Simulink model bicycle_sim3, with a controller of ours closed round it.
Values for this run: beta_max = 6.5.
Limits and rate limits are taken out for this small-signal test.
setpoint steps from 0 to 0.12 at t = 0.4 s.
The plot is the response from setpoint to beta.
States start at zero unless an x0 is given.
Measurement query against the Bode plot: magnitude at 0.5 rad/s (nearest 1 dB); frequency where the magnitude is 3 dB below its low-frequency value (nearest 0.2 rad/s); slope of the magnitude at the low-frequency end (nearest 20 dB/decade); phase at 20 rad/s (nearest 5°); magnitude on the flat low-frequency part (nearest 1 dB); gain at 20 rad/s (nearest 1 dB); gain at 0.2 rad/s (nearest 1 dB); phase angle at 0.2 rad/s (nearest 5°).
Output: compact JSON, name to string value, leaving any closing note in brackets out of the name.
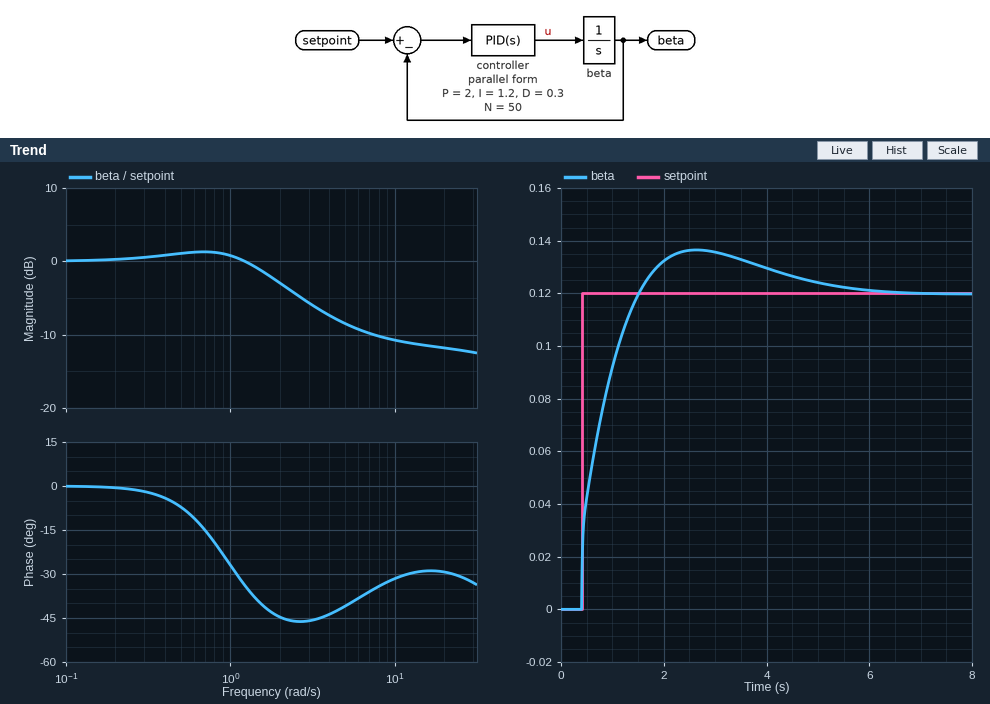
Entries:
{"magnitude at 0.5 rad/s": "1 dB", "frequency where the magnitude is 3 dB below its low-frequency value": "2.0 rad/s", "slope of the magnitude at the low-frequency end": "0 dB/decade", "phase at 20 rad/s": "-30°", "magnitude on the flat low-frequency part": "0 dB", "gain at 20 rad/s": "-12 dB", "gain at 0.2 rad/s": "0 dB", "phase angle at 0.2 rad/s": "0°"}
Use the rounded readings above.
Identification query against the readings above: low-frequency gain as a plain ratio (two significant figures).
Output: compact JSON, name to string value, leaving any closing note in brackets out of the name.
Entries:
{"low-frequency gain as a plain ratio": "1.0"}
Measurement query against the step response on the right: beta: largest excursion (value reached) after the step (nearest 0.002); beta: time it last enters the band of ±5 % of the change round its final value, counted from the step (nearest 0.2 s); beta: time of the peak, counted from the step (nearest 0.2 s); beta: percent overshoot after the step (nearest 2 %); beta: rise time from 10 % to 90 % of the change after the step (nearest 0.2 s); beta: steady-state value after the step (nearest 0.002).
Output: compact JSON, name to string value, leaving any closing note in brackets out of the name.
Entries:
{"beta: largest excursion (value reached) after the step": "0.136", "beta: time it last enters the band of ±5 % of the change round its final value, counted from the step": "4.2 s", "beta: time of the peak, counted from the step": "2.2 s", "beta: percent overshoot after the step": "14 %", "beta: rise time from 10 % to 90 % of the change after the step": "0.8 s", "beta: steady-state value after the step": "0.120"}
